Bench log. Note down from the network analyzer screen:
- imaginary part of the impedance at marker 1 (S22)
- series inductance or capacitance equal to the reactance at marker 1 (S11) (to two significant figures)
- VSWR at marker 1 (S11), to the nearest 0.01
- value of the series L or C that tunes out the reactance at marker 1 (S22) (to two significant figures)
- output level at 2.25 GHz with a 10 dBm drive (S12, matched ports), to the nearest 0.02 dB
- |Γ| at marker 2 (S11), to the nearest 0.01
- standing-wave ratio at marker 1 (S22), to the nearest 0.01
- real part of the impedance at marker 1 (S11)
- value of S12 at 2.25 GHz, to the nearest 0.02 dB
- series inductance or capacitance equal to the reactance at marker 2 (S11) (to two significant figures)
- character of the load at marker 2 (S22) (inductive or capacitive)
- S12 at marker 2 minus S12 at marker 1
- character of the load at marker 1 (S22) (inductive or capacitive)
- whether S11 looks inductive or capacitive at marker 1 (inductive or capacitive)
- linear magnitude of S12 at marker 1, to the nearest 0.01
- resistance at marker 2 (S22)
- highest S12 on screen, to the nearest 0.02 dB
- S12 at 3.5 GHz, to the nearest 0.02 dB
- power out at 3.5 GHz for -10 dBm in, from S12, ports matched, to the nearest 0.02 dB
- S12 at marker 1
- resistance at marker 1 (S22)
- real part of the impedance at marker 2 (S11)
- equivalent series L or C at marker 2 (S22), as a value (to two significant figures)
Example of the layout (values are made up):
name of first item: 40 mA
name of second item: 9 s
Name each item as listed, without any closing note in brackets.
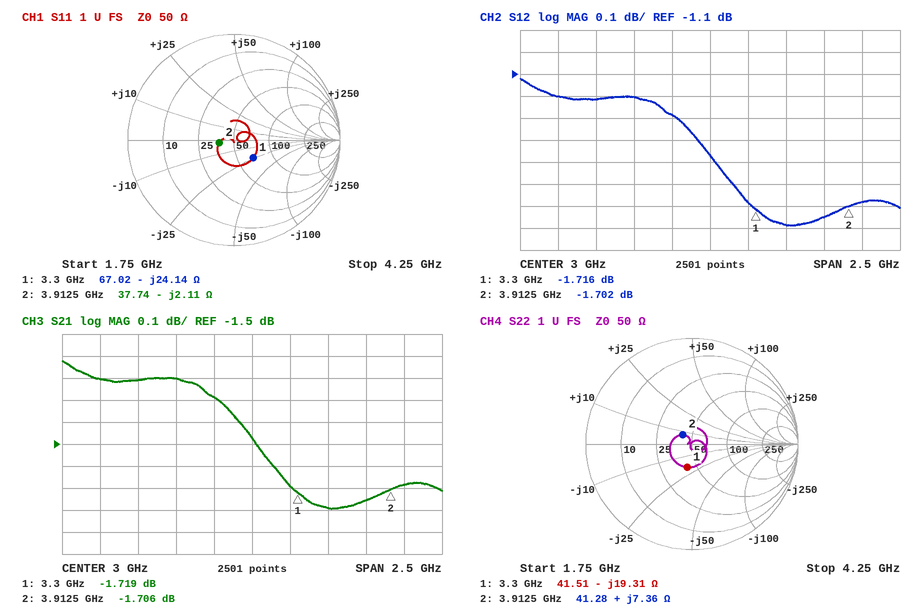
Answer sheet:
imaginary part of the impedance at marker 1: -19.31 Ω
series inductance or capacitance equal to the reactance at marker 1 (S11): 2.0 pF
VSWR at marker 1 (S11), to the nearest 0.01: 1.66
value of the series L or C that tunes out the reactance at marker 1 (S22): 930 pH
output level at 2.25 GHz with a 10 dBm drive (S12, matched ports), to the nearest 0.02 dB: 8.78 dBm
|Γ| at marker 2 (S11), to the nearest 0.01: 0.14
standing-wave ratio at marker 1 (S22), to the nearest 0.01: 1.58
real part of the impedance at marker 1: 67.02 Ω
value of S12 at 2.25 GHz, to the nearest 0.02 dB: -1.22 dB
series inductance or capacitance equal to the reactance at marker 2 (S11): 19 pF
character of the load at marker 2 (S22): inductive
S12 at marker 2 minus S12 at marker 1: 0.014 dB
character of the load at marker 1 (S22): capacitive
whether S11 looks inductive or capacitive at marker 1: capacitive
linear magnitude of S12 at marker 1, to the nearest 0.01: 0.82
resistance at marker 2: 41.28 Ω
highest S12 on screen, to the nearest 0.02 dB: -1.12 dB
S12 at 3.5 GHz, to the nearest 0.02 dB: -1.78 dB
power out at 3.5 GHz for -10 dBm in, from S12, ports matched, to the nearest 0.02 dB: -11.78 dBm
S12 at marker 1: -1.716 dB
resistance at marker 1: 41.51 Ω
real part of the impedance at marker 2: 37.74 Ω
equivalent series L or C at marker 2 (S22), as a value: 300 pH
